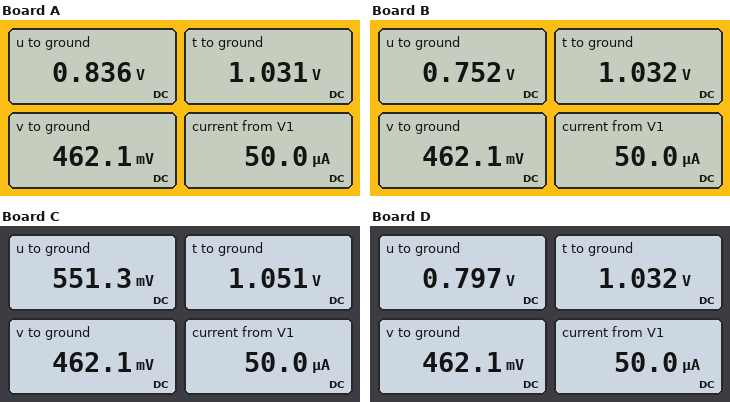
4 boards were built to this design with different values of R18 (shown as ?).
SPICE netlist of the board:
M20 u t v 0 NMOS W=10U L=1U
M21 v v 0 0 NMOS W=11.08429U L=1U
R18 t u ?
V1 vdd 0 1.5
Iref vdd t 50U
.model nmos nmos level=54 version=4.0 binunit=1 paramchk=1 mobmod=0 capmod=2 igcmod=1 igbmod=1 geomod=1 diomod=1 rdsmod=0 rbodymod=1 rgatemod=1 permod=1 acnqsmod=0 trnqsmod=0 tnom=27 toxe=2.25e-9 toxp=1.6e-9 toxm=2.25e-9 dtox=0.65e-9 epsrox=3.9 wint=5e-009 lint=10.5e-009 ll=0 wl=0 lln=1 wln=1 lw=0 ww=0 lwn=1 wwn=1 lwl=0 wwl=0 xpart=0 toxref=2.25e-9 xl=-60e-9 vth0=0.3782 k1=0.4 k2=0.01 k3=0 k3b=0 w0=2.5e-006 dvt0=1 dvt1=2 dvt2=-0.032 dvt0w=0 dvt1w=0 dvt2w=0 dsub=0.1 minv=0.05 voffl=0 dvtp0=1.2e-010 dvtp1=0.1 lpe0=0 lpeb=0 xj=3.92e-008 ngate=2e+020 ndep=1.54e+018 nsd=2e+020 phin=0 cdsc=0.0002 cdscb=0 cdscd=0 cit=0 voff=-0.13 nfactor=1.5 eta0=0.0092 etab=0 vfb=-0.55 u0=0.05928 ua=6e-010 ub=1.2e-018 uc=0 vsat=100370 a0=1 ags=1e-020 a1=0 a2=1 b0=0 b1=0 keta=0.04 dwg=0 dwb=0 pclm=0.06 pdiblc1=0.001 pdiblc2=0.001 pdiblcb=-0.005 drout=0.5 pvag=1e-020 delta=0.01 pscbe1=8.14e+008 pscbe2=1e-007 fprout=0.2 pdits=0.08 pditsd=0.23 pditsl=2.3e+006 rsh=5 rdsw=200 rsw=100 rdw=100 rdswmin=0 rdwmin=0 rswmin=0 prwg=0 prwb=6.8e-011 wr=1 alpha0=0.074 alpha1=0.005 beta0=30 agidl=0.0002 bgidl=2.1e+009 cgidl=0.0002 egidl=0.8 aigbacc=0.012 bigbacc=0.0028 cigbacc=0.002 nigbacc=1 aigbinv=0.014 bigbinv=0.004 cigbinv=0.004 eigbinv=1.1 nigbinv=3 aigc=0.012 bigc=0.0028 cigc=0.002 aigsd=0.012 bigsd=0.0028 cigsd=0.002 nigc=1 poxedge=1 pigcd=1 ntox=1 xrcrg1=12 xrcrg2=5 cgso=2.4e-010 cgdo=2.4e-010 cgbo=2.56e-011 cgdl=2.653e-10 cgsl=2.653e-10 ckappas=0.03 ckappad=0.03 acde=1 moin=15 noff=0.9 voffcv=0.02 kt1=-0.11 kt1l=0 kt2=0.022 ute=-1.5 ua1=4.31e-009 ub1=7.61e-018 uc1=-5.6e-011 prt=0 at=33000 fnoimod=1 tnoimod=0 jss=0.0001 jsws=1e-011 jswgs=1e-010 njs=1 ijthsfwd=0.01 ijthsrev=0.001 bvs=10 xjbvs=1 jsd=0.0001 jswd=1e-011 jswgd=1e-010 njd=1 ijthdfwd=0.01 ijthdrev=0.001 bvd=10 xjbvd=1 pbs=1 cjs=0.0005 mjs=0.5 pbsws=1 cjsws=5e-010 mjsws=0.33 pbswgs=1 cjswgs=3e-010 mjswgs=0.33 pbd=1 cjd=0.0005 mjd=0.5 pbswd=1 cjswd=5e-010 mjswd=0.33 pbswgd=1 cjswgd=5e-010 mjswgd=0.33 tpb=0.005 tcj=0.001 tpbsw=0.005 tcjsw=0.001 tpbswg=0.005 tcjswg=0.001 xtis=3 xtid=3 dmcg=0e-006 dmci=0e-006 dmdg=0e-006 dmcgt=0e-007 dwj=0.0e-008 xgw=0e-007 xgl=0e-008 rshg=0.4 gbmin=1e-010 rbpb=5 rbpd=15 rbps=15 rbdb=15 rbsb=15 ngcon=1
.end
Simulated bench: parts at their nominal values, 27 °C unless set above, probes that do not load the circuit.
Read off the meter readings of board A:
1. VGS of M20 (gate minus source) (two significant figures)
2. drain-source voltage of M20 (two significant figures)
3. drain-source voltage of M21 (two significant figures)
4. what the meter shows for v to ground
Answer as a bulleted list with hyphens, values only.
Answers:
- 570 mV
- 370 mV
- 460 mV
- 462.1 mV
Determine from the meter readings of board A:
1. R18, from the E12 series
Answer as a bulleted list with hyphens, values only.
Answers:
- 3.9 kΩ
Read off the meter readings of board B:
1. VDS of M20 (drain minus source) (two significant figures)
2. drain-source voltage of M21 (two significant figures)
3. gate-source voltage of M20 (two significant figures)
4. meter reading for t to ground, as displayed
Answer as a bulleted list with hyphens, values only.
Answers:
- 290 mV
- 460 mV
- 570 mV
- 1.032 V
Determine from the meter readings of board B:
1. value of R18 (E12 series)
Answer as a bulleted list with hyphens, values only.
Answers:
- 5.6 kΩ
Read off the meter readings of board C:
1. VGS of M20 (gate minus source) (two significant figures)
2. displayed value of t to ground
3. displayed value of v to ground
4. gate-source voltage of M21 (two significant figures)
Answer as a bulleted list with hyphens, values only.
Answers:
- 590 mV
- 1.051 V
- 462.1 mV
- 460 mV
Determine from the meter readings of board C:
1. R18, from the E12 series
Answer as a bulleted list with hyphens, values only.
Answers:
- 10 kΩ
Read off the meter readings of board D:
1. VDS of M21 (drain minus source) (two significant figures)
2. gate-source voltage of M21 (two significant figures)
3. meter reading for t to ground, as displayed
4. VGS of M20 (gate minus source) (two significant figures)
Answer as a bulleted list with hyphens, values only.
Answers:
- 460 mV
- 460 mV
- 1.032 V
- 570 mV
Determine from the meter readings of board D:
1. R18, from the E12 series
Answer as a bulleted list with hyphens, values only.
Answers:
- 4.7 kΩ
